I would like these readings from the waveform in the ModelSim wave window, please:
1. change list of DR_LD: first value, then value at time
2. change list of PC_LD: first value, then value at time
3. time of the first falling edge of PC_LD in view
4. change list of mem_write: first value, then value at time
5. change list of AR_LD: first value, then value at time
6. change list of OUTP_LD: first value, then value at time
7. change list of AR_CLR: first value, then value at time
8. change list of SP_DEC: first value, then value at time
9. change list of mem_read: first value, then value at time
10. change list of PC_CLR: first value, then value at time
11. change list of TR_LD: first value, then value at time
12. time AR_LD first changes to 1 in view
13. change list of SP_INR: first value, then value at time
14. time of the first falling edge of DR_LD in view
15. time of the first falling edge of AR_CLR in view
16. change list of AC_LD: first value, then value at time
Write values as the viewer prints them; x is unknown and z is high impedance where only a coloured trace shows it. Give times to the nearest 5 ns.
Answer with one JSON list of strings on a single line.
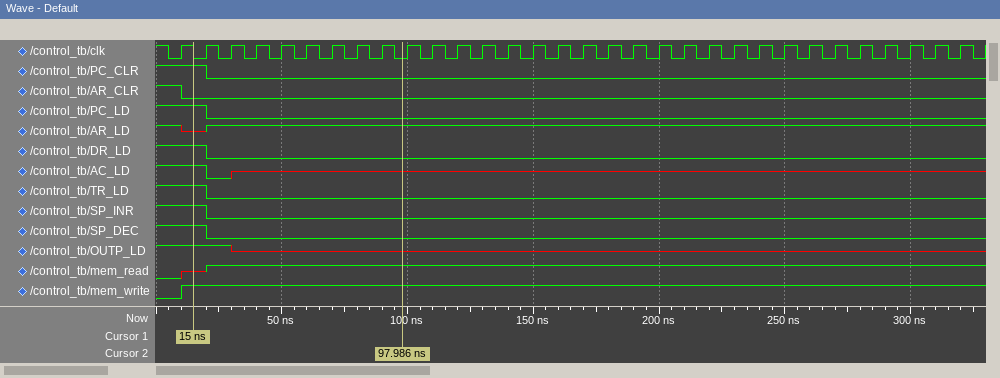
["1, 0 at 20 ns", "1, 0 at 20 ns", "20 ns", "0, 1 at 10 ns", "1, x at 10 ns, 1 at 20 ns", "1, x at 30 ns", "1, 0 at 10 ns", "1, 0 at 20 ns", "0, x at 10 ns, 1 at 20 ns", "1, 0 at 20 ns", "1, 0 at 20 ns", "20 ns", "1, 0 at 20 ns", "20 ns", "10 ns", "1, 0 at 20 ns, x at 30 ns"]
